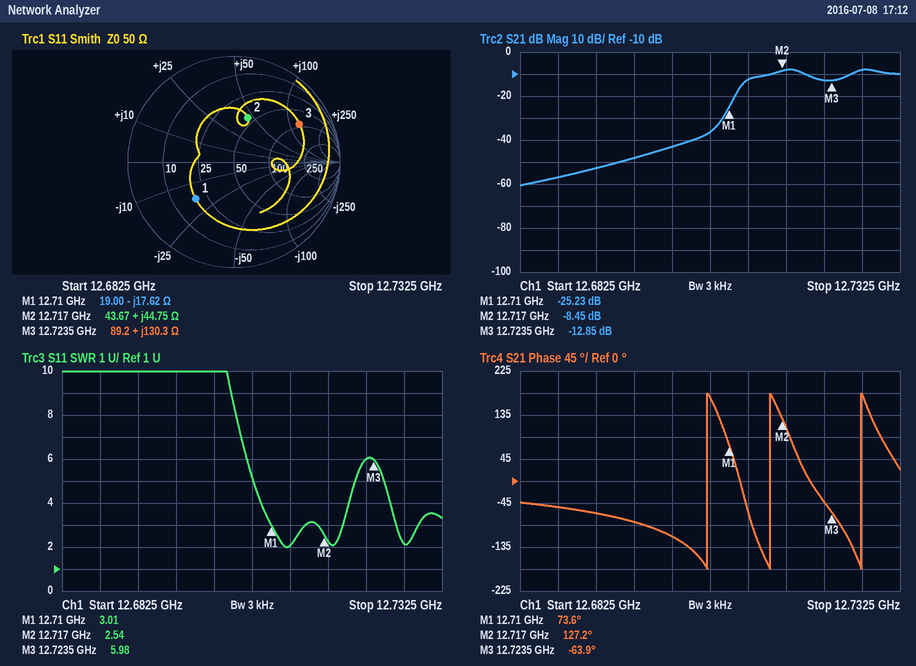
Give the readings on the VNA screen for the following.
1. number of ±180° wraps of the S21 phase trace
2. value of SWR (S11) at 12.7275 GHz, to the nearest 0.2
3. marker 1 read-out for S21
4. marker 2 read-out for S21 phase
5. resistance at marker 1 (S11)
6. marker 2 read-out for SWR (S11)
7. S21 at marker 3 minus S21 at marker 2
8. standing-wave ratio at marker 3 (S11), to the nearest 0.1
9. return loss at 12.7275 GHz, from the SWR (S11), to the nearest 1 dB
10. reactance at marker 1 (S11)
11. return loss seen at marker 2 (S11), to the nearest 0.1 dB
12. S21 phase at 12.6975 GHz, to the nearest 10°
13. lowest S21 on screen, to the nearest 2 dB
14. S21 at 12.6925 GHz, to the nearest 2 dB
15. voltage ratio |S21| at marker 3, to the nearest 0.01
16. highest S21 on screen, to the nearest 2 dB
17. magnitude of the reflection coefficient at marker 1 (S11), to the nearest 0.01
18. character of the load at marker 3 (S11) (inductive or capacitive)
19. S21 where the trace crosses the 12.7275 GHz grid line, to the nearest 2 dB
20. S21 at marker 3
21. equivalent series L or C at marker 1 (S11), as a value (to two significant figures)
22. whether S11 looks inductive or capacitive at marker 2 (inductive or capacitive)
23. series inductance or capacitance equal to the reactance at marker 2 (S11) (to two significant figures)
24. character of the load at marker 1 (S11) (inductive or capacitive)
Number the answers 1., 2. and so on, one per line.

1. 3
2. 2.2
3. -25.23 dB
4. 127.2°
5. 19.00 Ω
6. 2.54
7. -4.40 dB
8. 6.0
9. 9 dB
10. -17.62 Ω
11. 7.2 dB
12. -80°
13. -60 dB
14. -52 dB
15. 0.23
16. -8 dB
17. 0.50
18. inductive
19. -8 dB
20. -12.85 dB
21. 710 fF
22. inductive
23. 560 pH
24. capacitive
